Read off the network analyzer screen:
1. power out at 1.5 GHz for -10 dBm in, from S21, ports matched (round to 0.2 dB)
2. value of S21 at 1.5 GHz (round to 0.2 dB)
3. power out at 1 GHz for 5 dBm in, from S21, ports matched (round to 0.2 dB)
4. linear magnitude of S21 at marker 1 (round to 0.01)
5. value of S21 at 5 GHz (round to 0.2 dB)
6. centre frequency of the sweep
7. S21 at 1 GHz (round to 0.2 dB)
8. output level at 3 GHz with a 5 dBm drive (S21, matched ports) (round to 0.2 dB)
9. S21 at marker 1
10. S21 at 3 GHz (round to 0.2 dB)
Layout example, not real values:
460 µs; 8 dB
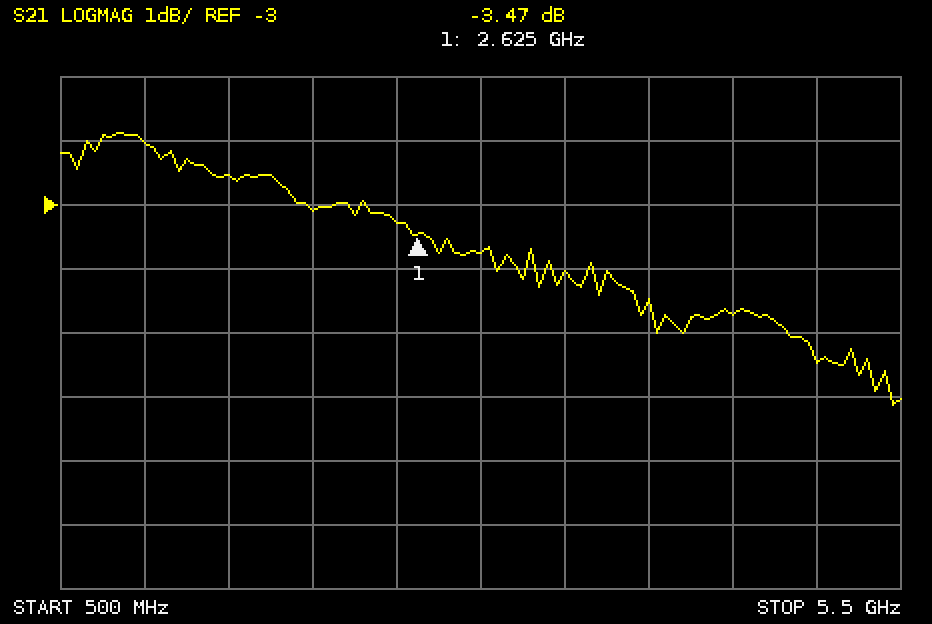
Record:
-12.6 dBm; -2.6 dB; 3.0 dBm; 0.67; -5.4 dB; 3 GHz; -2.0 dB; 1.2 dBm; -3.47 dB; -3.8 dB
